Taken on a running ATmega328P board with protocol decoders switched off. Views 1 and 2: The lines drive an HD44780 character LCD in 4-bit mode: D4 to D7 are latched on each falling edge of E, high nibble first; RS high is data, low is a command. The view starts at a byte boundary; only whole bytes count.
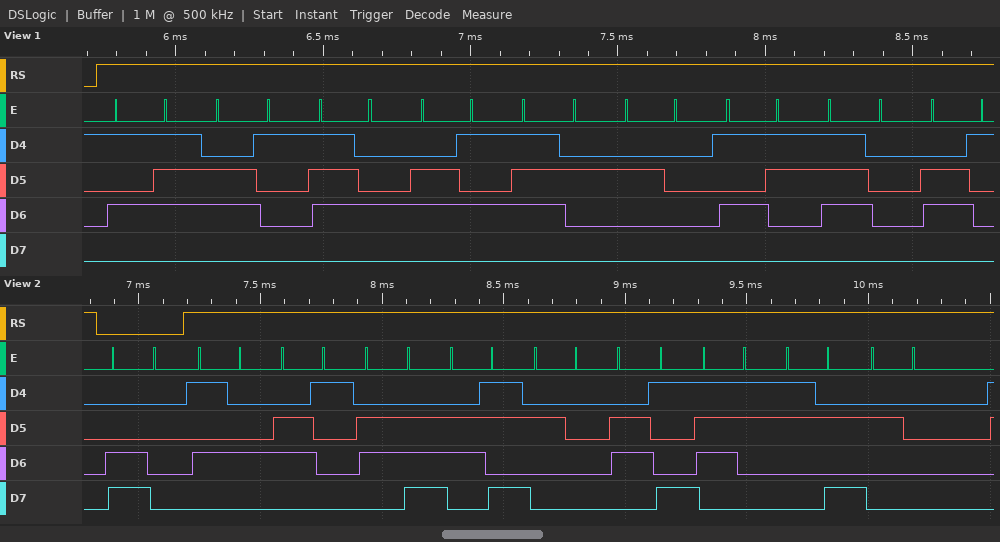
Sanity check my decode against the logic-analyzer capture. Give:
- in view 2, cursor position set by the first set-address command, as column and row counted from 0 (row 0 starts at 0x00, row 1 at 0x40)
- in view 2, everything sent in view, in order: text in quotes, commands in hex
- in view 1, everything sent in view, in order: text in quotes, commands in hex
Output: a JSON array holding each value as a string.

["column 0, row 1", "0xC0 \"Tank is: \"", "\"Water Spa\""]
